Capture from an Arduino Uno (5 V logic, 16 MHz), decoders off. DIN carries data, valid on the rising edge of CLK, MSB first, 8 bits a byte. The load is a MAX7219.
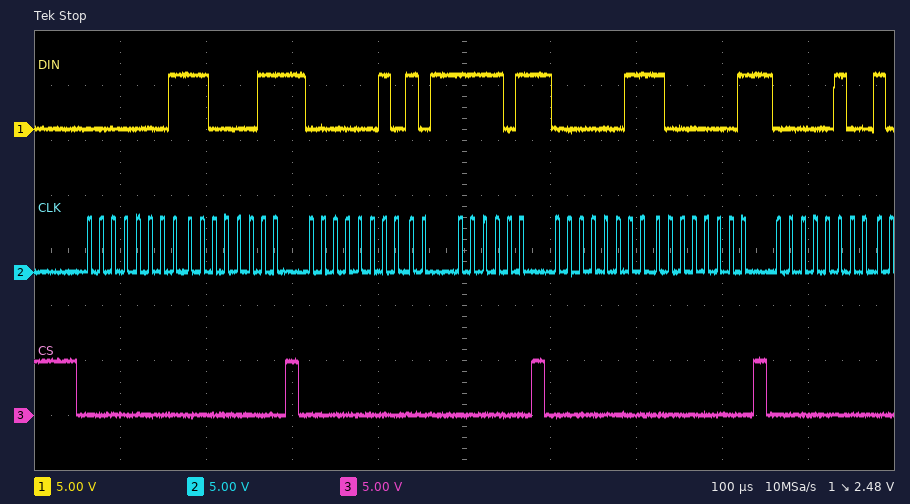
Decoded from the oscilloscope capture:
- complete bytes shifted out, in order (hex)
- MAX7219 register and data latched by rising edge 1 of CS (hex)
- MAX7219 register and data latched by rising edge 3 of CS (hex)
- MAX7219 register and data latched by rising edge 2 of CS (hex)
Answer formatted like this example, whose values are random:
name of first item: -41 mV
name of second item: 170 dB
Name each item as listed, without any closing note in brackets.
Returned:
complete bytes shifted out, in order: 01 C3 02 BD 03 81 04
MAX7219 register and data latched by rising edge 1 of CS: register 0x1, data 0xC3
MAX7219 register and data latched by rising edge 3 of CS: register 0x3, data 0x81
MAX7219 register and data latched by rising edge 2 of CS: register 0x2, data 0xBD
